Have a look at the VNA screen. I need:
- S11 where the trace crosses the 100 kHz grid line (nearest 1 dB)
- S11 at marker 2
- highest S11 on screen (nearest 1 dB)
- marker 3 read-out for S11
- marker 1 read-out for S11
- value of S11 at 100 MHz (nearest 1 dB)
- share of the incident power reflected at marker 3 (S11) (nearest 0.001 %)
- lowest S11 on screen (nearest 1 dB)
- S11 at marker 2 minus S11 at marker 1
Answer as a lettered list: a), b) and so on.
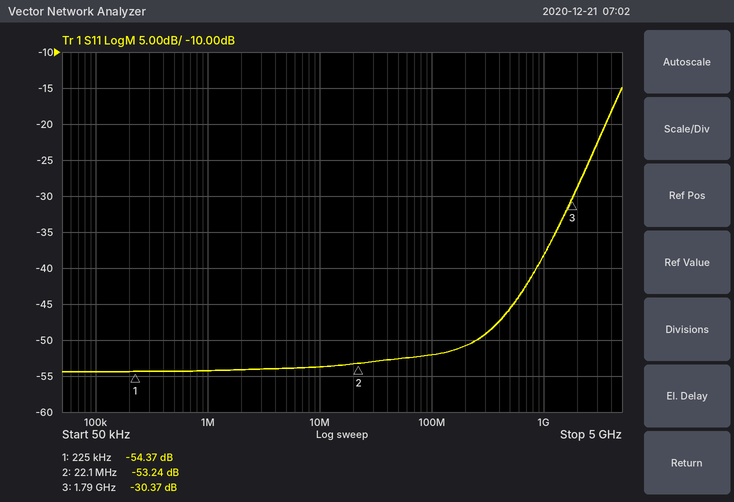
a) -54 dB
b) -53.24 dB
c) -15 dB
d) -30.37 dB
e) -54.37 dB
f) -52 dB
g) 0.092 %
h) -54 dB
i) 1.13 dB
